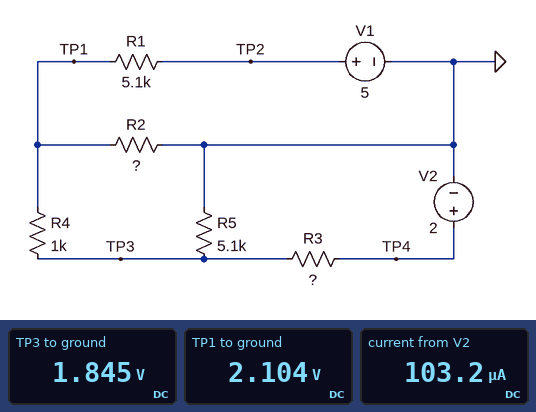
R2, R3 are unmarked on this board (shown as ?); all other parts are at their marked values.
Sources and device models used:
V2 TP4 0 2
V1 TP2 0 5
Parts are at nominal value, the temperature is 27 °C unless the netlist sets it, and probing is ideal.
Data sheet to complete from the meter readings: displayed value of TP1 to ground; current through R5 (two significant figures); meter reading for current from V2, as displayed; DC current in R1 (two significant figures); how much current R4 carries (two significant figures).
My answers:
2.104 V
360 µA
103.2 µA
570 µA
260 µA
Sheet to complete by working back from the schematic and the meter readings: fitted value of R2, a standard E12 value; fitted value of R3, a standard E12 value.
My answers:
6.8 kΩ
1.5 kΩ
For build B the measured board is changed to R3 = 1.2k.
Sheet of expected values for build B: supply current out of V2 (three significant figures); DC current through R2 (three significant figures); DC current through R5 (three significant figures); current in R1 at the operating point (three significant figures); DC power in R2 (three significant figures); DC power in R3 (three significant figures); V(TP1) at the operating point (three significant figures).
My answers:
112 µA
312 µA
366 µA
565 µA
660 µW
15.1 µW
2.12 V
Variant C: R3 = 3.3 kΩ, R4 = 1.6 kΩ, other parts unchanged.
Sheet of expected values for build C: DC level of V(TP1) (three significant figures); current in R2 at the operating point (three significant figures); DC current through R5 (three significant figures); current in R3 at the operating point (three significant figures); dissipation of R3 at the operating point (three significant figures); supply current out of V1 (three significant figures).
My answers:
2.12 V
312 µA
337 µA
85.1 µA
23.9 µW
564 µA
